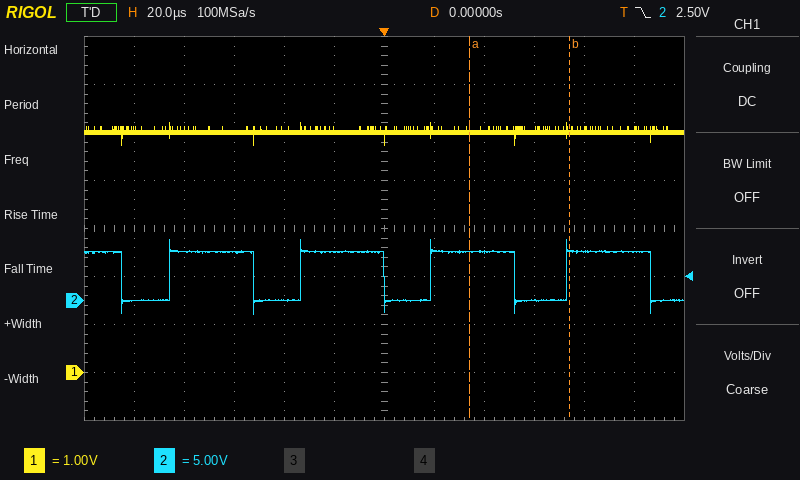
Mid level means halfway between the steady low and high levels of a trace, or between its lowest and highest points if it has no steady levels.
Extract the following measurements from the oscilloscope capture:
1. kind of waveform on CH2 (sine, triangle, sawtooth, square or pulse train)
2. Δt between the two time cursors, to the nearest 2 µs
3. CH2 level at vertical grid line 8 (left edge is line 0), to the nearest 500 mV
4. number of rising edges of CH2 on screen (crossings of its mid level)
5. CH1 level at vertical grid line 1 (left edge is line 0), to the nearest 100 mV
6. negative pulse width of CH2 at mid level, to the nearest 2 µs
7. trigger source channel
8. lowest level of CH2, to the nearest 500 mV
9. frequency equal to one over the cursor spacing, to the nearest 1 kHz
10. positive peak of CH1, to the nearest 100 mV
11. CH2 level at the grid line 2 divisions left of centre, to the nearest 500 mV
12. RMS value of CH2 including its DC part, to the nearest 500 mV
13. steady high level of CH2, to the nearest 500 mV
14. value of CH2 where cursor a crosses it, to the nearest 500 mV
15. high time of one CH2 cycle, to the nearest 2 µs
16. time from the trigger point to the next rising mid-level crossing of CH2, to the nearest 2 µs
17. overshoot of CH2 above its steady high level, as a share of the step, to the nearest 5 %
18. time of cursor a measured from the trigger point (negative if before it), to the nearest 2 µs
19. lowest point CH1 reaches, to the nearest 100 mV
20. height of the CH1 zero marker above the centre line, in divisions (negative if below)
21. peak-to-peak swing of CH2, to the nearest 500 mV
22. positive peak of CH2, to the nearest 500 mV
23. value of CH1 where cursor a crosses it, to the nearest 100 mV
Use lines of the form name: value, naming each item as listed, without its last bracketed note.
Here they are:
kind of waveform on CH2: pulse train
Δt between the two time cursors, to the nearest 2 µs: 40 µs
CH2 level at vertical grid line 8 (left edge is line 0), to the nearest 500 mV: 5.0 V
number of rising edges of CH2 on screen: 4
CH1 level at vertical grid line 1 (left edge is line 0), to the nearest 100 mV: 5.0 V
negative pulse width of CH2 at mid level, to the nearest 2 µs: 20 µs
trigger source channel: CH2
lowest level of CH2, to the nearest 500 mV: -1.5 V
frequency equal to one over the cursor spacing, to the nearest 1 kHz: 25 kHz
positive peak of CH1, to the nearest 100 mV: 5.2 V
CH2 level at the grid line 2 divisions left of centre, to the nearest 500 mV: 0.0 V
RMS value of CH2 including its DC part, to the nearest 500 mV: 4.0 V
steady high level of CH2, to the nearest 500 mV: 5.0 V
value of CH2 where cursor a crosses it, to the nearest 500 mV: 5.0 V
high time of one CH2 cycle, to the nearest 2 µs: 34 µs
time from the trigger point to the next rising mid-level crossing of CH2, to the nearest 2 µs: 18 µs
overshoot of CH2 above its steady high level, as a share of the step, to the nearest 5 %: 25 %
time of cursor a measured from the trigger point (negative if before it), to the nearest 2 µs: +34 µs
lowest point CH1 reaches, to the nearest 100 mV: 4.7 V
height of the CH1 zero marker above the centre line, in divisions: -3.0 div
peak-to-peak swing of CH2, to the nearest 500 mV: 8.0 V
positive peak of CH2, to the nearest 500 mV: 6.5 V
value of CH1 where cursor a crosses it, to the nearest 100 mV: 5.0 V
